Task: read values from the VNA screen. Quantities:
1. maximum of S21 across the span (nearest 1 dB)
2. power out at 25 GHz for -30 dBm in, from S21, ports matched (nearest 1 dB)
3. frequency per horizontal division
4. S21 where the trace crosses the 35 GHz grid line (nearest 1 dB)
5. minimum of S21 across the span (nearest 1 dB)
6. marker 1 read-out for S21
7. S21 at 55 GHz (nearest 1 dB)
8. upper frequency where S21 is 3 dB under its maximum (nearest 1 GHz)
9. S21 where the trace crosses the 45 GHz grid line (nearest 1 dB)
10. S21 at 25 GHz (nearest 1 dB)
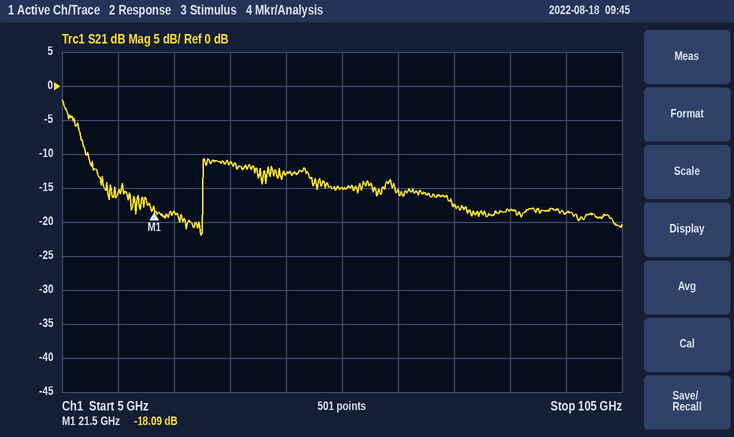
-2 dB
-48 dBm
10 GHz
-11 dB
-22 dB
-18.09 dB
-15 dB
7 GHz
-13 dB
-18 dB
